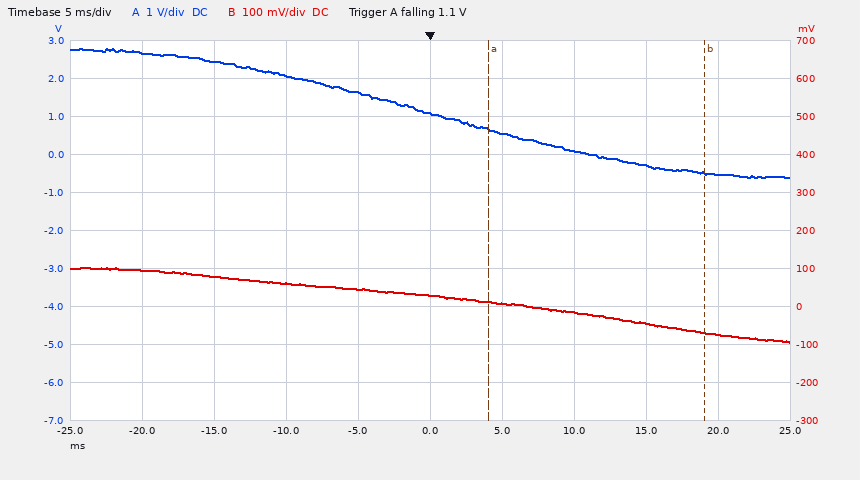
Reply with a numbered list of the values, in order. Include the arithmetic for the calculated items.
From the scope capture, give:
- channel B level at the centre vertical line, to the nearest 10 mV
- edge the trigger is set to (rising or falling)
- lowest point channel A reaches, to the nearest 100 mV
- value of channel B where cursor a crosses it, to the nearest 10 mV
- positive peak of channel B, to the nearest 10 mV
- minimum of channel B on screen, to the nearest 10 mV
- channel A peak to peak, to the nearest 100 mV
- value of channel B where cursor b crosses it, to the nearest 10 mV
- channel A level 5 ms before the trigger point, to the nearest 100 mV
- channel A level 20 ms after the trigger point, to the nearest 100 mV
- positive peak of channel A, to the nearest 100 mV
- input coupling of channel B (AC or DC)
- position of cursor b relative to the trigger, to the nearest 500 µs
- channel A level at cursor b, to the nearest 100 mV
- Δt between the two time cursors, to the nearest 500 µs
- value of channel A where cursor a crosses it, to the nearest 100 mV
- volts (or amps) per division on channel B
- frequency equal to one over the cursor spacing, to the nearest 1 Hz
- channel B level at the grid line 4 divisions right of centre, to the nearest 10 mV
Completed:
1. 30 mV
2. falling
3. -600 mV
4. 10 mV
5. 100 mV
6. -90 mV
7. 2.8 V − (-600 mV) = 3.4 V
8. -70 mV
9. 1.6 V
10. -500 mV
11. 2.8 V
12. DC
13. +19.0 ms
14. -500 mV
15. 15.0 ms
16. 700 mV
17. 100 mV
18. 1 / 15.0 ms ≈ 67 Hz
19. -70 mV
